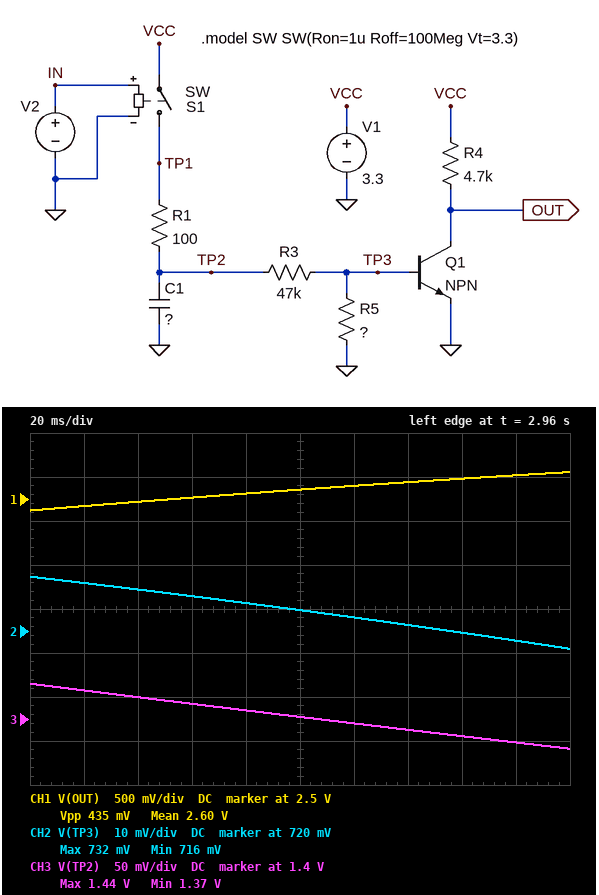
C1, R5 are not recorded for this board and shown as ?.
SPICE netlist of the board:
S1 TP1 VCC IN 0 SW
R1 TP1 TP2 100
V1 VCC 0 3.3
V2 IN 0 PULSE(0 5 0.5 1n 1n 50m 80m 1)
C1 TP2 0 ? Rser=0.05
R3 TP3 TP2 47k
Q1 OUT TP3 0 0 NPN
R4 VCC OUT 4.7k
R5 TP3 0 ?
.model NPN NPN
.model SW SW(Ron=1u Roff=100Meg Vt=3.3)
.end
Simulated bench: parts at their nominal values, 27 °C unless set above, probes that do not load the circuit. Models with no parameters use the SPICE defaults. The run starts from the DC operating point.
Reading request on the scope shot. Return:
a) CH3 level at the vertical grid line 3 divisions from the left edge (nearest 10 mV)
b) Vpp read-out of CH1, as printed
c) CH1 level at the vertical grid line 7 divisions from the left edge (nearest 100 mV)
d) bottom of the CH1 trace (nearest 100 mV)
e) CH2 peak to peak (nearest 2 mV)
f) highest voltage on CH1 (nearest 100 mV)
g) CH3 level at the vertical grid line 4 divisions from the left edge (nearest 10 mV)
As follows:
1.42 V
435 mV
2.7 V
2.4 V
16 mV
2.8 V
1.41 V
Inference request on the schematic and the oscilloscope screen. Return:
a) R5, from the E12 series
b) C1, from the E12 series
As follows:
56 kΩ
39 µF
